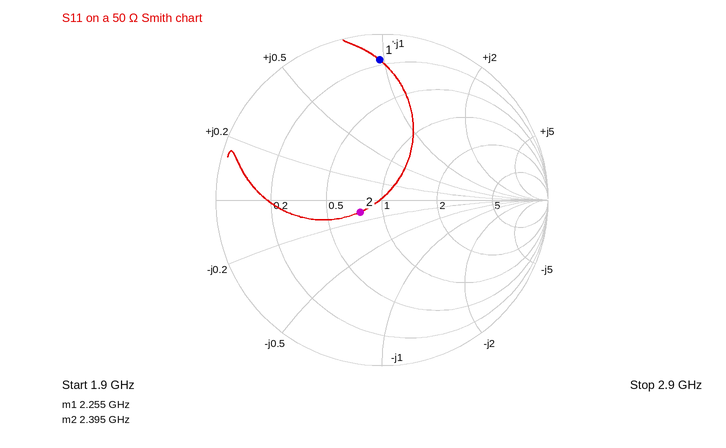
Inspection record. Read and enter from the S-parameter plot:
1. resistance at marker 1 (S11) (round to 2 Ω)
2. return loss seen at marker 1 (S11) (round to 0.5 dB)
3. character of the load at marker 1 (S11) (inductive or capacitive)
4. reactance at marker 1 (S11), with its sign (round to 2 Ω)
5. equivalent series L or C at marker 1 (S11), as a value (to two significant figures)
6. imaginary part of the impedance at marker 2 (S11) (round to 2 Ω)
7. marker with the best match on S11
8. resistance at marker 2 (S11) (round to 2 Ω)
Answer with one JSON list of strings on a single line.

["8 Ω", "1.5 dB", "inductive", "+48 Ω", "3.4 nH", "-6 Ω", "marker 2", "38 Ω"]
